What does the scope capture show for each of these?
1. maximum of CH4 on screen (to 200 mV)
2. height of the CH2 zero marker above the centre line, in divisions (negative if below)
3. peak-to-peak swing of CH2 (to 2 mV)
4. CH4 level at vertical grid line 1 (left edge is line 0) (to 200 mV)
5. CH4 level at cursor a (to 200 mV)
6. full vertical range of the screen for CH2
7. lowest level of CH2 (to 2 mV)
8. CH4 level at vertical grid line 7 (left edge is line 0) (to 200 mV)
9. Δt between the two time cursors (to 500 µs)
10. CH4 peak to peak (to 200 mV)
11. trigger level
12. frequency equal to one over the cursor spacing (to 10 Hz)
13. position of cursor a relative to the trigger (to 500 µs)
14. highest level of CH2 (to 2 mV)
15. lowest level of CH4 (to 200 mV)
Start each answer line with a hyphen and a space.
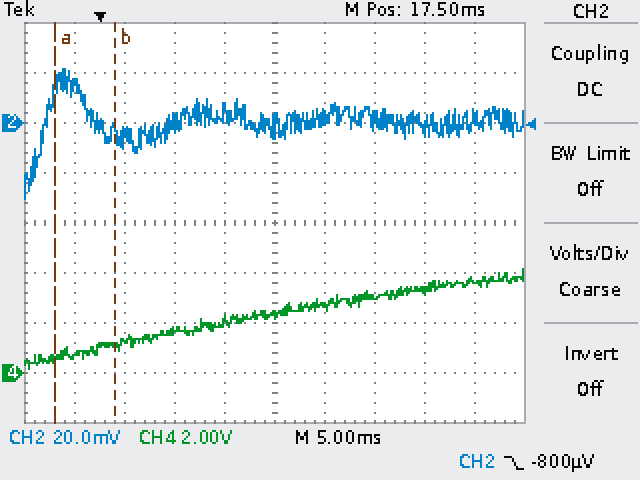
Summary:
- 4.2 V
- +2.0 div
- 52 mV
- 800 mV
- 600 mV
- 160 mV
- -30 mV
- 3.0 V
- 6.0 ms
- 4.0 V
- -800 µV
- 170 Hz
- -4.5 ms
- 22 mV
- 200 mV
